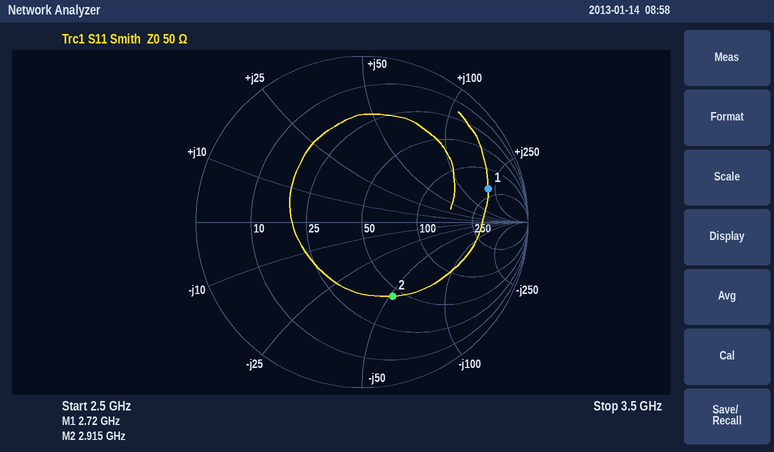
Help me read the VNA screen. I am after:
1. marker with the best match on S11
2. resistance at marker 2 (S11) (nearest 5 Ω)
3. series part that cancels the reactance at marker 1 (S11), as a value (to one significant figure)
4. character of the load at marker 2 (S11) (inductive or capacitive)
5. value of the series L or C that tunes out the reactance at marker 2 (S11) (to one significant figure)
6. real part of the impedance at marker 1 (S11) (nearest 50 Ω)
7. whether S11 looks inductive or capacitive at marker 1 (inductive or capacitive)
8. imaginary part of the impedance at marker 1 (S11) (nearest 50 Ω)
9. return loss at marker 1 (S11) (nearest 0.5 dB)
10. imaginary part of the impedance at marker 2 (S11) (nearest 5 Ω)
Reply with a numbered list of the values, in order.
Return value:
1. marker 2
2. 45 Ω
3. 300 fF
4. capacitive
5. 3 nH
6. 200 Ω
7. inductive
8. +200 Ω
9. 2.0 dB
10. -50 Ω
